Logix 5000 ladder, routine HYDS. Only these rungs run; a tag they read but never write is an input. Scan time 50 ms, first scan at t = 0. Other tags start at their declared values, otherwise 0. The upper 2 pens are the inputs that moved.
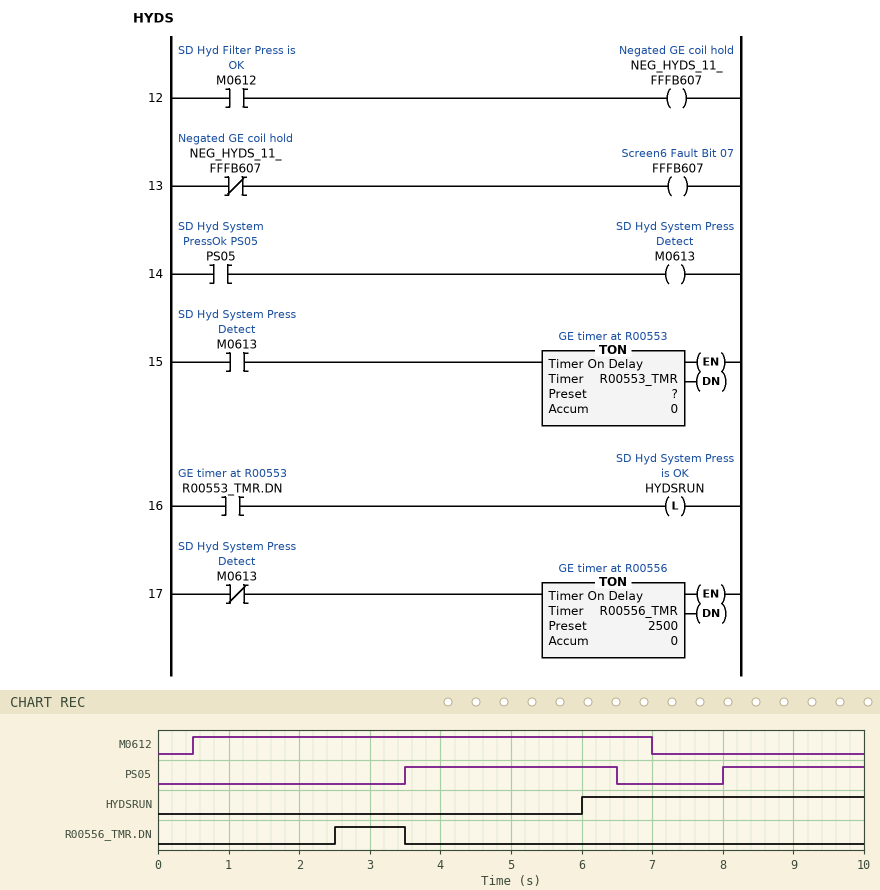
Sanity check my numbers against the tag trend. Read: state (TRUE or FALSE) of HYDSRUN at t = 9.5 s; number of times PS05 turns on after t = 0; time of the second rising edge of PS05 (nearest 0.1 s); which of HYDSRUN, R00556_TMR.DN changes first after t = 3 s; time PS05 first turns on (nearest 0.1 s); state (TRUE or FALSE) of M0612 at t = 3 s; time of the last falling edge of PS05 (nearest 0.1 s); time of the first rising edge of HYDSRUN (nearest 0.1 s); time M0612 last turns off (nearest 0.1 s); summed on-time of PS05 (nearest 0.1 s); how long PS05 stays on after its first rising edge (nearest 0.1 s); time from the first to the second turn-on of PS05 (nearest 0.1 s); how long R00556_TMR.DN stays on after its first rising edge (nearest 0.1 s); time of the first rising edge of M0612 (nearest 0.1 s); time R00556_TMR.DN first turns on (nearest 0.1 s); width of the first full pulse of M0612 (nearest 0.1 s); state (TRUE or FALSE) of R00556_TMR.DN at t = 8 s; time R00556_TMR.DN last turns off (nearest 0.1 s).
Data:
TRUE
2
8.0 s
R00556_TMR.DN
3.5 s
TRUE
6.5 s
6.0 s
7.0 s
5.0 s
3.0 s
4.5 s
1.0 s
0.5 s
2.5 s
6.5 s
FALSE
3.5 s
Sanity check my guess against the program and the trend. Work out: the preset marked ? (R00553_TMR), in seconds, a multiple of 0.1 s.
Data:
2.5 s
